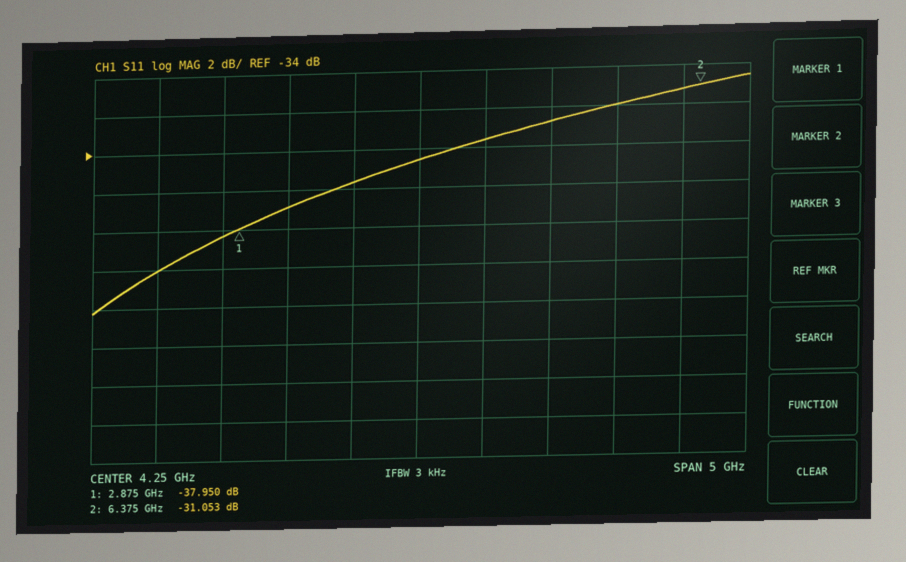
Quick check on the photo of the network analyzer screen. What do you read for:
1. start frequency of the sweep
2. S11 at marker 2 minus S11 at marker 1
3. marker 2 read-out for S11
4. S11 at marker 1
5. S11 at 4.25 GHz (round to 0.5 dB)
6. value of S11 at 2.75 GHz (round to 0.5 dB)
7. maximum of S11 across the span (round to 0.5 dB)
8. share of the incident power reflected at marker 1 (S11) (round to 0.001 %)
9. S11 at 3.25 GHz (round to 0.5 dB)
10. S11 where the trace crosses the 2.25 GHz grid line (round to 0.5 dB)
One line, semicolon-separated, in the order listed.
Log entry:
1.75 GHz; 6.897 dB; -31.053 dB; -37.950 dB; -34.5 dB; -38.5 dB; -30.5 dB; 0.016 %; -37.0 dB; -40.0 dB
